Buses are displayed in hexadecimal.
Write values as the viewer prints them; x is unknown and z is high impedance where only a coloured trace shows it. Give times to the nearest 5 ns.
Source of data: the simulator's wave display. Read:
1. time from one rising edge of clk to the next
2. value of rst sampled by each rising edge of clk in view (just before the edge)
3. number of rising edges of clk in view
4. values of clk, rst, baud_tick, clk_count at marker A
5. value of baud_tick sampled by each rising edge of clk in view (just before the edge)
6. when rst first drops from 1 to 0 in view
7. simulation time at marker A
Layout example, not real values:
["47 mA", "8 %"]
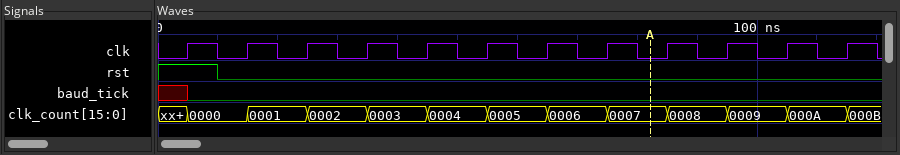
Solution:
["10 ns", "1 0 0 0 0 0 0 0 0 0 0 0", "12", "clk=0, rst=0, baud_tick=0, clk_count=0007", "x 0 0 0 0 0 0 0 0 0 0 0", "10 ns", "80 ns"]
